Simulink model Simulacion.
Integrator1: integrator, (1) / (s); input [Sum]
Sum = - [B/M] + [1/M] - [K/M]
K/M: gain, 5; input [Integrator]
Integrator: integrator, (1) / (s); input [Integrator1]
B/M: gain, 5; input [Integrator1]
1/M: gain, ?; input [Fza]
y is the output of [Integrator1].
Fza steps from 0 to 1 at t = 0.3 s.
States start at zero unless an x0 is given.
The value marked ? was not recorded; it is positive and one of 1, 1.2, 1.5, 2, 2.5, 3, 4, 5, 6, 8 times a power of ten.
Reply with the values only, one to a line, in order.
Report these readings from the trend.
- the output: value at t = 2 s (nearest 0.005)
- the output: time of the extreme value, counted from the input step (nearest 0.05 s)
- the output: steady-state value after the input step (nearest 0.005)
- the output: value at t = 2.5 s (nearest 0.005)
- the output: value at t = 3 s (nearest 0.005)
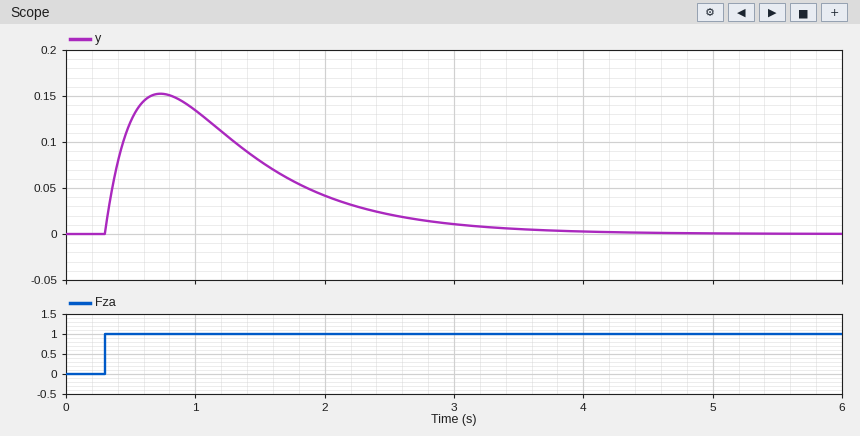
0.040
0.45 s
0.000
0.020
0.010
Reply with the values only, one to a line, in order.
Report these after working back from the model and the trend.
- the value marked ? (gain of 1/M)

1
